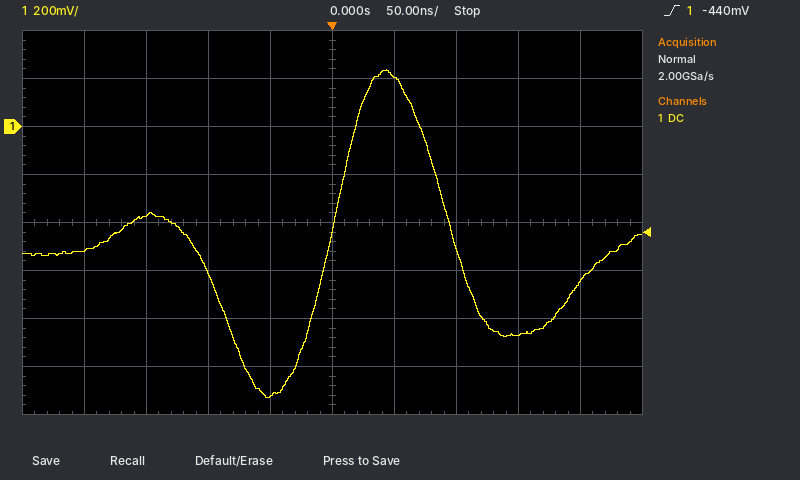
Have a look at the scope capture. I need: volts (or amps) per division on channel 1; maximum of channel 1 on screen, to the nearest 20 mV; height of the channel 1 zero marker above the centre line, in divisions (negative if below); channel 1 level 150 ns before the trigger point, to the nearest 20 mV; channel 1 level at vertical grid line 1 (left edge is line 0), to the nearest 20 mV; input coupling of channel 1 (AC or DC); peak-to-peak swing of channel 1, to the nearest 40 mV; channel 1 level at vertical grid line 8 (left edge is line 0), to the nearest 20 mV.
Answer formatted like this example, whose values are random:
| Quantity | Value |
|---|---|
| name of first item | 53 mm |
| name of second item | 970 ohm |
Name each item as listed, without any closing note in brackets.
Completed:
| Quantity | Value |
|---|---|
| volts (or amps) per division on channel 1 | 200 mV |
| maximum of channel 1 on screen, to the nearest 20 mV | 240 mV |
| height of the channel 1 zero marker above the centre line, in divisions | +2.0 div |
| channel 1 level 150 ns before the trigger point, to the nearest 20 mV | -360 mV |
| channel 1 level at vertical grid line 1 (left edge is line 0), to the nearest 20 mV | -520 mV |
| input coupling of channel 1 | DC |
| peak-to-peak swing of channel 1, to the nearest 40 mV | 1.36 V |
| channel 1 level at vertical grid line 8 (left edge is line 0), to the nearest 20 mV | -860 mV |
